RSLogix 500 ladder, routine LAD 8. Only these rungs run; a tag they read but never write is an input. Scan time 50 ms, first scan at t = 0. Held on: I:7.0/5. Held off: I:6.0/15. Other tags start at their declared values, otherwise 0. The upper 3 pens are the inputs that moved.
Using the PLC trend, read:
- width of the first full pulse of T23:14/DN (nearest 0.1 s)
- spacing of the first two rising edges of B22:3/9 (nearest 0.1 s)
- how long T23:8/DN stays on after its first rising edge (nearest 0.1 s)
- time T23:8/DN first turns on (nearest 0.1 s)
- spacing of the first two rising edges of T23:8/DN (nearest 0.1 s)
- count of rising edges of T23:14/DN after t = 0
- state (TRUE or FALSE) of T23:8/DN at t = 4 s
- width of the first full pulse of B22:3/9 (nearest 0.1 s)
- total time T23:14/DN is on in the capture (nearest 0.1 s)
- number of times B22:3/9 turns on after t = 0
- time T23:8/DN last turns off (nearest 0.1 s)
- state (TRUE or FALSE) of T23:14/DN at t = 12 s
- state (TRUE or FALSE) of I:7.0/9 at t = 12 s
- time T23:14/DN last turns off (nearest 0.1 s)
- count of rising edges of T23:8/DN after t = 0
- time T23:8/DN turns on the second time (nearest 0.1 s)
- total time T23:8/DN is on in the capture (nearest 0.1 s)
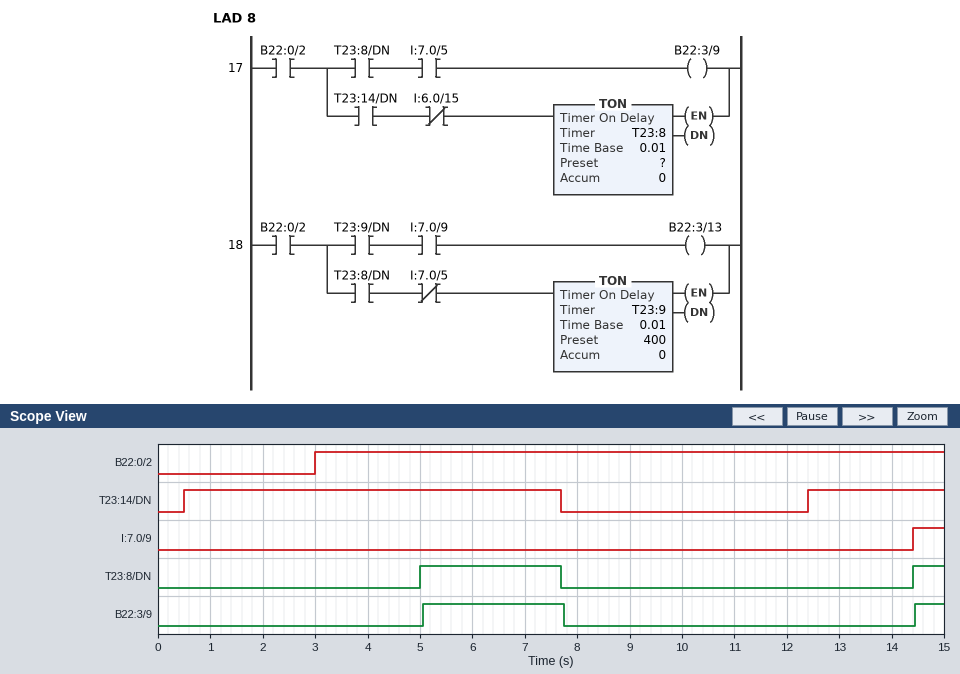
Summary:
7.2 s
9.4 s
2.7 s
5.0 s
9.4 s
2
FALSE
2.7 s
9.8 s
2
7.7 s
FALSE
FALSE
7.7 s
2
14.4 s
3.3 s
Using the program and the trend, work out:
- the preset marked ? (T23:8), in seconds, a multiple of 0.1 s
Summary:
2.0 s
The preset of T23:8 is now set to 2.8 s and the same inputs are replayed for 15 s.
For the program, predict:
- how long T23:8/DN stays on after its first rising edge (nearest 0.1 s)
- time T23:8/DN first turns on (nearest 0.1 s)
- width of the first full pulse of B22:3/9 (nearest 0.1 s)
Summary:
1.9 s
5.8 s
1.9 s
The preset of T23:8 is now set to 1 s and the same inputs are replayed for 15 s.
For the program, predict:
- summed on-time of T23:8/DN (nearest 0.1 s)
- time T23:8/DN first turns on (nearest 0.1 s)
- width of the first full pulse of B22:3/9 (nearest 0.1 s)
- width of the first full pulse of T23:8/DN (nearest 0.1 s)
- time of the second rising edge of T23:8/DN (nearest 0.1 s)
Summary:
5.3 s
4.0 s
3.7 s
3.7 s
13.4 s
